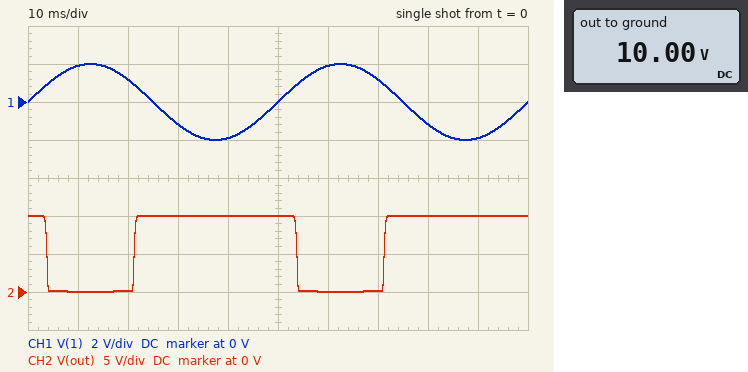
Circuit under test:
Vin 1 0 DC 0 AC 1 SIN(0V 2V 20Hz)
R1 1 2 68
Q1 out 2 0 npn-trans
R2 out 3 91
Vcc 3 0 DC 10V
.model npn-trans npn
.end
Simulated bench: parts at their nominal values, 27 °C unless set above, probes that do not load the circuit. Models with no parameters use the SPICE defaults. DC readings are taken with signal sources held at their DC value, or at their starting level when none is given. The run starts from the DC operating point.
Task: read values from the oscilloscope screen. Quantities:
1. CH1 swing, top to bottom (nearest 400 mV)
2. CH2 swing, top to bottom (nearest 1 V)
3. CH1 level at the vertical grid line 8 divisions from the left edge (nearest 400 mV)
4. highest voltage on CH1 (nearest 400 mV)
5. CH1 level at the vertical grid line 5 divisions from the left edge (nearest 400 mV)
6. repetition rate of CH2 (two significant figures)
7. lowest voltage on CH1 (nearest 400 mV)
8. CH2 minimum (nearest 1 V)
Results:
4.0 V
10 V
-1.2 V
2.0 V
0 V
20 Hz
-2.0 V
0 V
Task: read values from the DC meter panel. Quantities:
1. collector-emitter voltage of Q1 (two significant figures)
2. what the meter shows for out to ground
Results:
10 V
10.00 V
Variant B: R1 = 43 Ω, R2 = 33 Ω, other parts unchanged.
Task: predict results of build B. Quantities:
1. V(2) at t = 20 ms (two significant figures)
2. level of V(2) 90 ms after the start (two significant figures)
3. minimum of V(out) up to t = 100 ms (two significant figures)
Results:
920 mV
-1.9 V
72 mV
